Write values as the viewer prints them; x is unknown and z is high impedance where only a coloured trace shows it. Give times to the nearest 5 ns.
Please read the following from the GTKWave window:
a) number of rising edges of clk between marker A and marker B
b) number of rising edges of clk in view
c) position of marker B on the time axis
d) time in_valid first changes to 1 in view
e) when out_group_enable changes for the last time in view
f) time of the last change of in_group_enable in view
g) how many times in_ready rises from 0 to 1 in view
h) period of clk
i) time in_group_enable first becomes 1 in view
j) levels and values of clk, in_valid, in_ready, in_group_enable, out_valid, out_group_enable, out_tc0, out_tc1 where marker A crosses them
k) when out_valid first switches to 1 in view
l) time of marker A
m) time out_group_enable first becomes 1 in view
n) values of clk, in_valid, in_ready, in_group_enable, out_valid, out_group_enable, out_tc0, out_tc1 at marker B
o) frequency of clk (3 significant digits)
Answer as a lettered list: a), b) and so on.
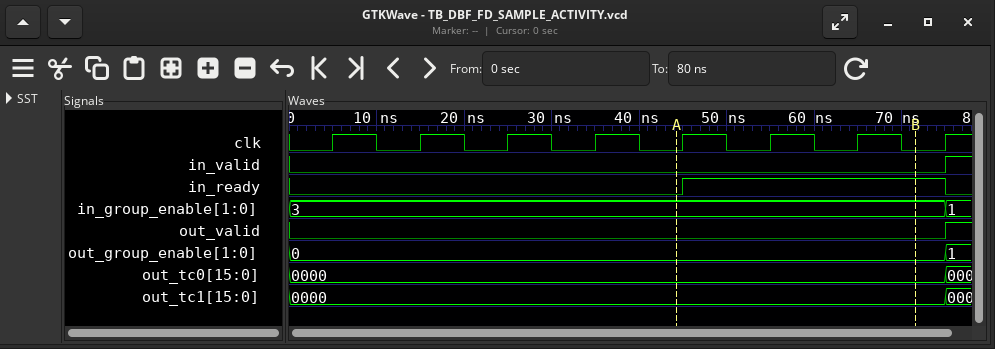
a) 3
b) 8
c) 70 ns
d) 75 ns
e) 75 ns
f) 75 ns
g) 1
h) 10 ns
i) 75 ns
j) clk=0, in_valid=0, in_ready=0, in_group_enable=3, out_valid=0, out_group_enable=0, out_tc0=0000, out_tc1=0000
k) 75 ns
l) 45 ns
m) 75 ns
n) clk=0, in_valid=0, in_ready=1, in_group_enable=3, out_valid=0, out_group_enable=0, out_tc0=0000, out_tc1=0000
o) 100 MHz
